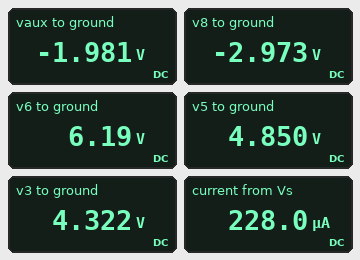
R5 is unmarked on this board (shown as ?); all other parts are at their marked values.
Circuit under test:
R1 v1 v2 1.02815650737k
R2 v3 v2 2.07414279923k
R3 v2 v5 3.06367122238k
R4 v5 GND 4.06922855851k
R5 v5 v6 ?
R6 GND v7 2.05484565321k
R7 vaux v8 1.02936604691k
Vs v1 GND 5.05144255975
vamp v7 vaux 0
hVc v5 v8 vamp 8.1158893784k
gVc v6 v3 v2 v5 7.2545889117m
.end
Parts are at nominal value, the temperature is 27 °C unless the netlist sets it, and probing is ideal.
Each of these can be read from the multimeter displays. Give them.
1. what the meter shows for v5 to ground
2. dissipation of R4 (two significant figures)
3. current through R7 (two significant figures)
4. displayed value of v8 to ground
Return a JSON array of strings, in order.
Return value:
["4.850 V", "5.8 mW", "960 µA", "-2.973 V"]
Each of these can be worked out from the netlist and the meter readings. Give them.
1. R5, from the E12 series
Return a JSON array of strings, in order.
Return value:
["5.6 kΩ"]
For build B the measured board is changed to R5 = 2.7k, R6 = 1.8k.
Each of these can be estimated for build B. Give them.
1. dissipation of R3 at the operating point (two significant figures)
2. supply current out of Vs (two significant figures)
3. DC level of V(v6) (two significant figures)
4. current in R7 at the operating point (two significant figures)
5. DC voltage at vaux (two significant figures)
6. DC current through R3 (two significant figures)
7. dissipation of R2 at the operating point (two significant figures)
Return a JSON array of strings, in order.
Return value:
["500 nW", "270 µA", "5.6 V", "910 µA", "-1.6 V", "13 µA", "170 µW"]
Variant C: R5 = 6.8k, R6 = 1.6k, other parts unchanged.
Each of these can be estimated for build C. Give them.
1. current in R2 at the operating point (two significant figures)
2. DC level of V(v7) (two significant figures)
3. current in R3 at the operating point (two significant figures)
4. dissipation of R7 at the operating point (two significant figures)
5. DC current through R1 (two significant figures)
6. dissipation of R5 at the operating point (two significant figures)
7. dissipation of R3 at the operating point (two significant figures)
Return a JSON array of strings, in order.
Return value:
["320 µA", "-1.4 V", "14 µA", "780 µW", "300 µA", "690 µW", "630 nW"]
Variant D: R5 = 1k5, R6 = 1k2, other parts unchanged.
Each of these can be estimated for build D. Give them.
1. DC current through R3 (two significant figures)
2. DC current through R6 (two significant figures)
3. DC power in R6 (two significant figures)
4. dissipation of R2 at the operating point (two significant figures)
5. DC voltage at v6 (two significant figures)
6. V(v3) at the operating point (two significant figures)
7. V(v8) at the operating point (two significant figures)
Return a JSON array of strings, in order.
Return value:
["17 µA", "800 µA", "780 µW", "290 µW", "5.3 V", "3.9 V", "-1.8 V"]
